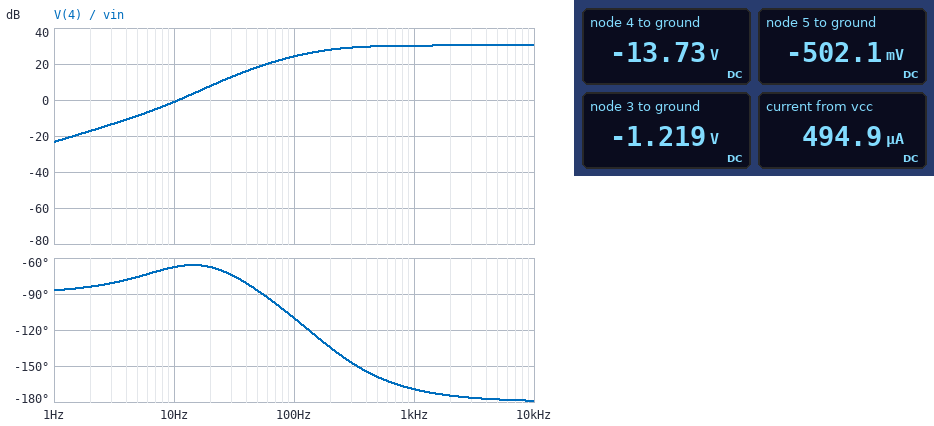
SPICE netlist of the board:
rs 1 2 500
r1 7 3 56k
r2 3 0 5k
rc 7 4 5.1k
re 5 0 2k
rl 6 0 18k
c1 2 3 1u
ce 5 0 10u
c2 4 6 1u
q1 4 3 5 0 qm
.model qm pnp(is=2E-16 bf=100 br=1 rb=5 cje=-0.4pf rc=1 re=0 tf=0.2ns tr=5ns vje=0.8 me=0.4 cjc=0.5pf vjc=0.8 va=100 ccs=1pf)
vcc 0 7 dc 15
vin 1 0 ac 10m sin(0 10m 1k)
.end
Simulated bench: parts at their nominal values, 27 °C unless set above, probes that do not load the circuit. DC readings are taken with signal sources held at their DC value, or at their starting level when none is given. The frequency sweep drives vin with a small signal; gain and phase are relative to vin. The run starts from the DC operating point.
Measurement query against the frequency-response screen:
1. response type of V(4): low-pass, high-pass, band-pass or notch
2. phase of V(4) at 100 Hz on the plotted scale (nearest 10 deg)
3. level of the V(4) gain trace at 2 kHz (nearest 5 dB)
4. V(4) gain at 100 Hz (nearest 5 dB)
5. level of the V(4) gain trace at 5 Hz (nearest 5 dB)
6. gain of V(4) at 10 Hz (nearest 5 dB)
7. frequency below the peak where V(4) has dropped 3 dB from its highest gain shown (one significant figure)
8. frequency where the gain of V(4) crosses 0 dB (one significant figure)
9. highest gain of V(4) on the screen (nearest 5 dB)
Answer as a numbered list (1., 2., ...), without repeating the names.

1. high-pass
2. -110 deg
3. 30 dB
4. 25 dB
5. -10 dB
6. 0 dB
7. 200 Hz
8. 10 Hz
9. 30 dB
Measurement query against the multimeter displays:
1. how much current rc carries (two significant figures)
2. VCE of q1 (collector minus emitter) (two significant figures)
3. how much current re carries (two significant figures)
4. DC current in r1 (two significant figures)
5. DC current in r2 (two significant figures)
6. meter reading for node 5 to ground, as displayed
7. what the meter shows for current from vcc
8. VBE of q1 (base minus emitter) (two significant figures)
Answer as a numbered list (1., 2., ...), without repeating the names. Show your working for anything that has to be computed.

1. (-13.73 V - (-15 V)) / 5.1 kΩ = 250 µA
2. -13.73 V - (-502.1 mV) = -13 V
3. (0 V - (-502.1 mV)) / 2 kΩ = 250 µA
4. (-1.219 V - (-15 V)) / 56 kΩ = 250 µA
5. (0 V - (-1.219 V)) / 5 kΩ = 240 µA
6. -502.1 mV
7. 494.9 µA
8. -1.219 V - (-502.1 mV) = -720 mV
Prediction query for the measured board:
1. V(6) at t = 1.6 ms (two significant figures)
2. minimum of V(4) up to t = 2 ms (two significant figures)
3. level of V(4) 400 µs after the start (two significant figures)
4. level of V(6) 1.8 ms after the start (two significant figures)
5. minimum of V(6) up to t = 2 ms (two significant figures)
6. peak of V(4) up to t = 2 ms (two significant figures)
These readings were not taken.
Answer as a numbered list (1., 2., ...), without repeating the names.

1. 260 mV
2. -14 V
3. -14 V
4. 310 mV
5. -280 mV
6. -13 V
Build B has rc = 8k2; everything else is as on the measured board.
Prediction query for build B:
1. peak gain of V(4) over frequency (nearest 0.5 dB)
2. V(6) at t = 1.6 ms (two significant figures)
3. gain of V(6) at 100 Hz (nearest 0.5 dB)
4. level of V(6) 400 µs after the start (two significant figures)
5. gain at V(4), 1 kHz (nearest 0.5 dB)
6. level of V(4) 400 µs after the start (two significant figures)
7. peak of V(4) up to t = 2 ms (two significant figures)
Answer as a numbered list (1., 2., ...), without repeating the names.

1. 33.5 dB
2. 360 mV
3. 27.0 dB
4. -140 mV
5. 33.0 dB
6. -13 V
7. -12 V
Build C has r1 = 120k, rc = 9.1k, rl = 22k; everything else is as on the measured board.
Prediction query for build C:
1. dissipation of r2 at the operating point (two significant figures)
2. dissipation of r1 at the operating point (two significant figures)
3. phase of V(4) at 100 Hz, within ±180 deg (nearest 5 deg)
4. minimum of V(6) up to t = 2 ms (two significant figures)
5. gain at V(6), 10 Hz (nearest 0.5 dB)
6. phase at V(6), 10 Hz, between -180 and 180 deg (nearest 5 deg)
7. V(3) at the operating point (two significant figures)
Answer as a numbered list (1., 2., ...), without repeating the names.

1. 72 µW
2. 1.7 mW
3. -165 deg
4. -4.2 mV
5. -17.5 dB
6. -75 deg
7. -600 mV
